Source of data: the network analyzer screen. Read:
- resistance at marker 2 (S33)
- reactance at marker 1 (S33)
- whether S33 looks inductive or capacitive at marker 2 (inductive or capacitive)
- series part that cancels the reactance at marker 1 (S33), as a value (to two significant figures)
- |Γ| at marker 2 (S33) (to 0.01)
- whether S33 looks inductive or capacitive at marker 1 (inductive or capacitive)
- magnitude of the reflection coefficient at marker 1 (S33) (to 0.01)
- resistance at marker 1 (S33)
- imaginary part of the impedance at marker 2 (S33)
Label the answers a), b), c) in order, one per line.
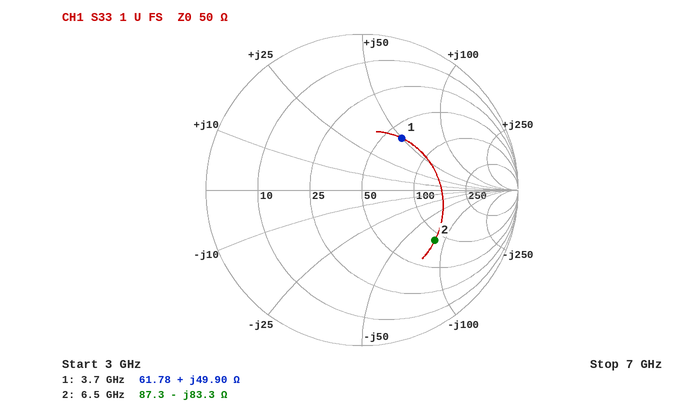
a) 87.3 Ω
b) +49.90 Ω
c) capacitive
d) 860 fF
e) 0.57
f) inductive
g) 0.42
h) 61.78 Ω
i) -83.3 Ω
